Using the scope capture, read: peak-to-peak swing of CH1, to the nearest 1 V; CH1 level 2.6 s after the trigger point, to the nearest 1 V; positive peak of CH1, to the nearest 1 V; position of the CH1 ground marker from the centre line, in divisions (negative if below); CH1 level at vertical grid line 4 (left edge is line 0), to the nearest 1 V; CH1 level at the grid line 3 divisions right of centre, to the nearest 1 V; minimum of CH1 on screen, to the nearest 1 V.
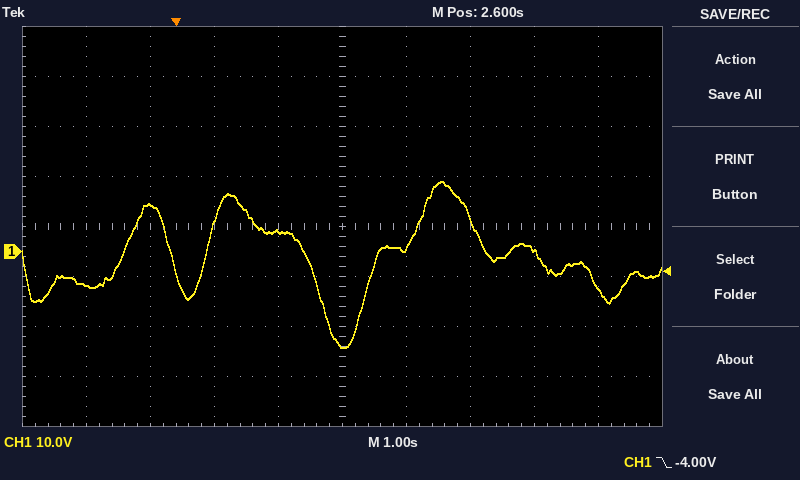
33 V
-19 V
14 V
-0.5 div
4 V
0 V
-19 V
